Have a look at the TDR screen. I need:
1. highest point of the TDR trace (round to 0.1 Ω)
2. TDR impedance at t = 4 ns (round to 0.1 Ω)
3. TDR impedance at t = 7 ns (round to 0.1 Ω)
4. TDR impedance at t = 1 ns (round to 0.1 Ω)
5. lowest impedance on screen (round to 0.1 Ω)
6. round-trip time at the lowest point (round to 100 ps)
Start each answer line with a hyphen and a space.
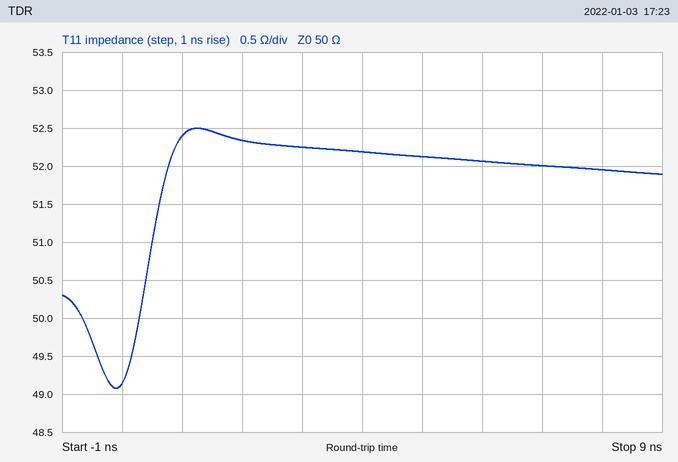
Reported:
- 52.5 Ω
- 52.2 Ω
- 52.0 Ω
- 52.4 Ω
- 49.1 Ω
- -100 ps
